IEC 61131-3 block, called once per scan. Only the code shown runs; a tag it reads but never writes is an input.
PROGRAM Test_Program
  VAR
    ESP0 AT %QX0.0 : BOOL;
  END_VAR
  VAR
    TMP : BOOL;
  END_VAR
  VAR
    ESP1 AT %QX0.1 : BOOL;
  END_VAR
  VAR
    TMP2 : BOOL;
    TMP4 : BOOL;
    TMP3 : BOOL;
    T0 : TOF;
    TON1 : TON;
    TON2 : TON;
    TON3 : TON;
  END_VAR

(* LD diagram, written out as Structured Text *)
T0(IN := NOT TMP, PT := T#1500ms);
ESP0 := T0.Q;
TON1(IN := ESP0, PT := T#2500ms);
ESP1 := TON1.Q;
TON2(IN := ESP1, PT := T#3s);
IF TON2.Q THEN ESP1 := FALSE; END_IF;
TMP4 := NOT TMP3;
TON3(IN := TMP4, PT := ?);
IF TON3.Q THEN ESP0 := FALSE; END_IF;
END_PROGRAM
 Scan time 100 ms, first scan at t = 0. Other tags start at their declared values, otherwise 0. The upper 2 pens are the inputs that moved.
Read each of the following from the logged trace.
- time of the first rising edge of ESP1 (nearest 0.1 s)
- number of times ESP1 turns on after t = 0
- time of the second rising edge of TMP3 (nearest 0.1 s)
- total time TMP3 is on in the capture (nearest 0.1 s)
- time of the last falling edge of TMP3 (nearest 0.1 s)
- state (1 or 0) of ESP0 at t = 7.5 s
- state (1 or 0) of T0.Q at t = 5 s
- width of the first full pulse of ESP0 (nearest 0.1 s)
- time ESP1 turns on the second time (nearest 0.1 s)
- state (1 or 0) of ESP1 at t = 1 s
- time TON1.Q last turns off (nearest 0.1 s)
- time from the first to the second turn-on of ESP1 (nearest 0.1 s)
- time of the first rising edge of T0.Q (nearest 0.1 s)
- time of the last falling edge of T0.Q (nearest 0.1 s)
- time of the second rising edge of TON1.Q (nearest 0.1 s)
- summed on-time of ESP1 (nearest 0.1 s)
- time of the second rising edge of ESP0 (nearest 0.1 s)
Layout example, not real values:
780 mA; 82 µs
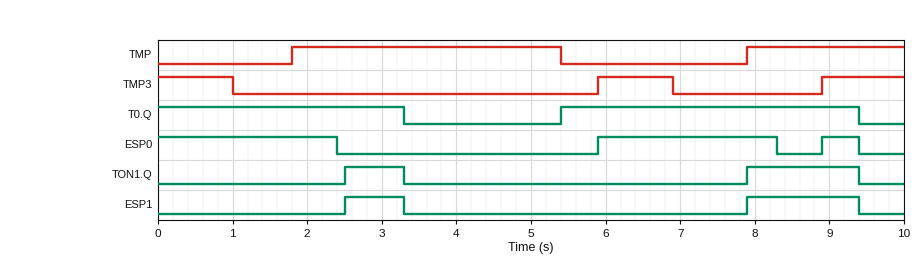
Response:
2.5 s; 2; 8.9 s; 3.1 s; 6.9 s; 1; 0; 2.4 s; 7.9 s; 0; 9.4 s; 5.4 s; 5.4 s; 9.4 s; 7.9 s; 2.3 s; 8.9 s
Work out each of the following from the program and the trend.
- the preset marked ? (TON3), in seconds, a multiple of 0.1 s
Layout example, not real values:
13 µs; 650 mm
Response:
1.4 s
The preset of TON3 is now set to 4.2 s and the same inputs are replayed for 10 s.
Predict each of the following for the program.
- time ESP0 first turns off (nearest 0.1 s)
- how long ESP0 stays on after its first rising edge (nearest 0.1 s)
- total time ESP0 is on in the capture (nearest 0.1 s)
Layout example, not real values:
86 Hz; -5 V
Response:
3.3 s; 3.5 s; 6.8 s
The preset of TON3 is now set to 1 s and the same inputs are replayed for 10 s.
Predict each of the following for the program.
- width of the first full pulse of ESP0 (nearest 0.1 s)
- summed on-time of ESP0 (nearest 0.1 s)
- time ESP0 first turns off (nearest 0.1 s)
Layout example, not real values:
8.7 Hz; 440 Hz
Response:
2.0 s; 4.5 s; 2.0 s
